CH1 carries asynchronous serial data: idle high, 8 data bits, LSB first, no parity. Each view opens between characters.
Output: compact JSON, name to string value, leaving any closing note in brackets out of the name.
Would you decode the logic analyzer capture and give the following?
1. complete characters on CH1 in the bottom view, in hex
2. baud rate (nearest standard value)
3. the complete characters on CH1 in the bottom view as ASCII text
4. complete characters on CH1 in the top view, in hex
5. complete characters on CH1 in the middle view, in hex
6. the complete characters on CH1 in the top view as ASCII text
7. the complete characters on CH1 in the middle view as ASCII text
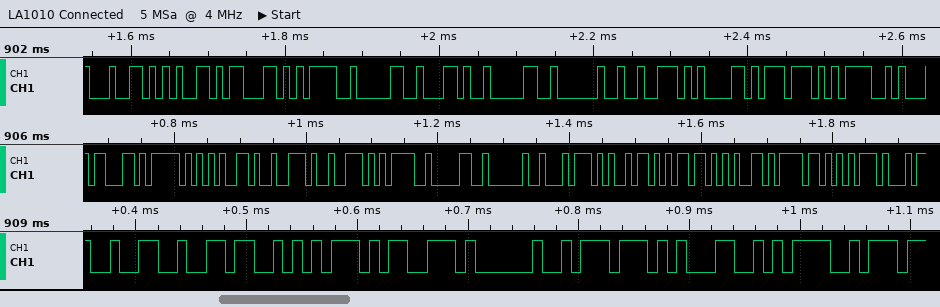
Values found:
{"complete characters on CH1 in the bottom view, in hex": "32, 36, 75, 73, 20, 77, 31, 3D", "baud rate": "115200 baud", "the complete characters on CH1 in the bottom view as ASCII text": "\"26us w1=\"", "complete characters on CH1 in the top view, in hex": "64, 65, 63, 3D, 30, 2C, 30, 20, 72, 61, 77, 3D", "complete characters on CH1 in the middle view, in hex": "63, 5F, 65, 72, 72, 3D, 30, 20, 74, 69, 6D, 65, 6F, 75", "the complete characters on CH1 in the top view as ASCII text": "\"dec=0,0 raw=\"", "the complete characters on CH1 in the middle view as ASCII text": "\"c_err=0 timeou\""}
